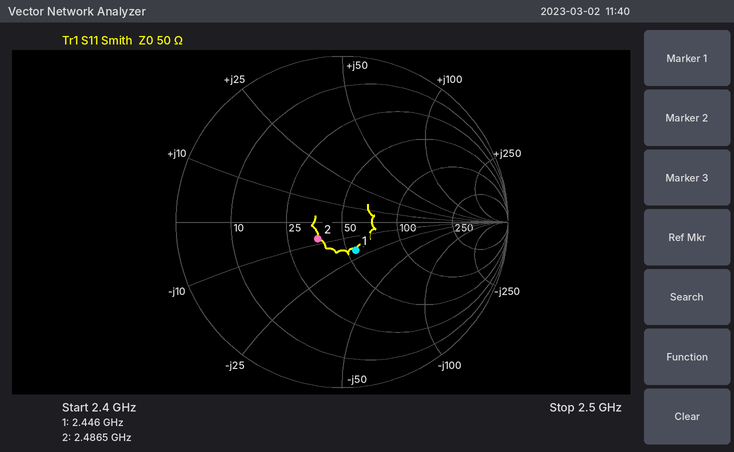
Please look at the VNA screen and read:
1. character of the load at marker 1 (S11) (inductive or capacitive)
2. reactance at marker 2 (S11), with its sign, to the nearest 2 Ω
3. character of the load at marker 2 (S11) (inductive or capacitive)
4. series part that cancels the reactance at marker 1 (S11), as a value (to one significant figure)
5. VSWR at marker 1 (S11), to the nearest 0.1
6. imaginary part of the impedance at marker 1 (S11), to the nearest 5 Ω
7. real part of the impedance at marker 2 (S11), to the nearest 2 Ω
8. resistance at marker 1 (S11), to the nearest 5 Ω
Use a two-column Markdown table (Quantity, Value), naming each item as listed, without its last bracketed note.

| Quantity | Value |
|---|---|
| character of the load at marker 1 (S11) | capacitive |
| reactance at marker 2 (S11), with its sign, to the nearest 2 Ω | -8 Ω |
| character of the load at marker 2 (S11) | capacitive |
| series part that cancels the reactance at marker 1 (S11), as a value | 1 nH |
| VSWR at marker 1 (S11), to the nearest 0.1 | 1.5 |
| imaginary part of the impedance at marker 1 (S11), to the nearest 5 Ω | -20 Ω |
| real part of the impedance at marker 2 (S11), to the nearest 2 Ω | 36 Ω |
| resistance at marker 1 (S11), to the nearest 5 Ω | 55 Ω |
